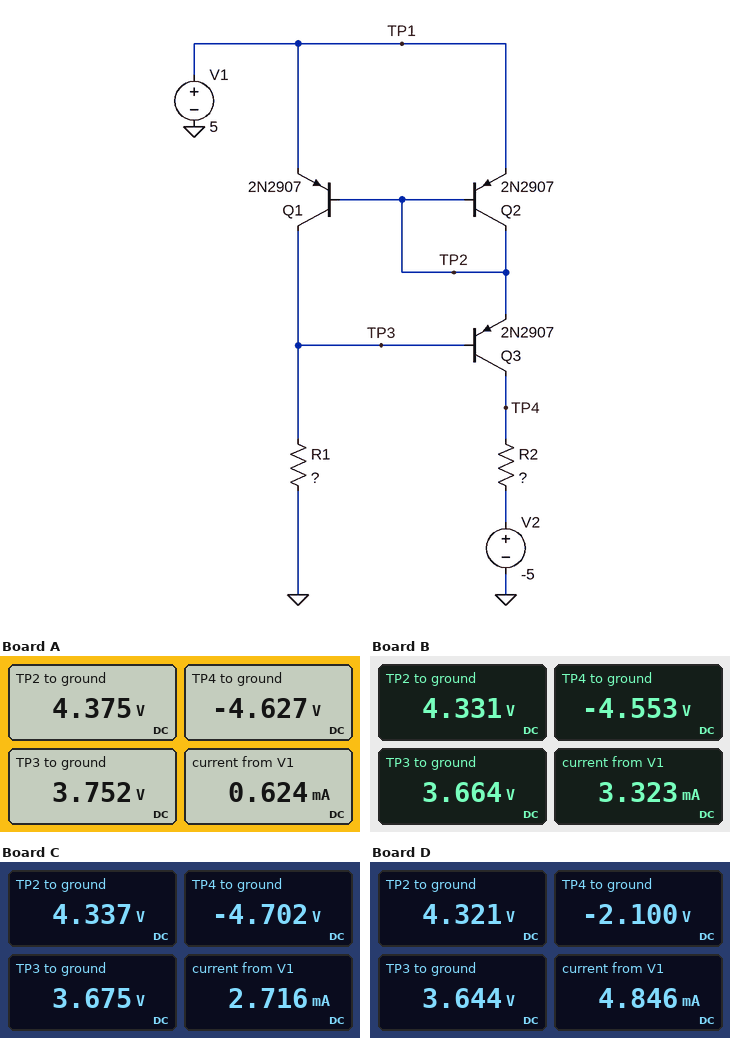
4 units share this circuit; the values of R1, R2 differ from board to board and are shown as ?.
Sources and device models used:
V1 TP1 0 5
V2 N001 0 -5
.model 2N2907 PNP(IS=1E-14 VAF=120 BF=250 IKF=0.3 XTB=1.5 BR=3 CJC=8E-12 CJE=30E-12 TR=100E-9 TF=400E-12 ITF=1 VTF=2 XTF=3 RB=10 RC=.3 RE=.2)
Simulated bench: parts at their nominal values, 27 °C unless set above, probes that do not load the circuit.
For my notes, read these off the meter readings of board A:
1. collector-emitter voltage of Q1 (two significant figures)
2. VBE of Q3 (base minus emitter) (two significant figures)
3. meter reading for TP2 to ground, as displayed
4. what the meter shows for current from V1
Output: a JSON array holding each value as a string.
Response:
["-1.2 V", "-620 mV", "4.375 V", "0.624 mA"]
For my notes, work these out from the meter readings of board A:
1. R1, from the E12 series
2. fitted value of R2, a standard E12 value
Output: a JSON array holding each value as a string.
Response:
["12 kΩ", "1.2 kΩ"]
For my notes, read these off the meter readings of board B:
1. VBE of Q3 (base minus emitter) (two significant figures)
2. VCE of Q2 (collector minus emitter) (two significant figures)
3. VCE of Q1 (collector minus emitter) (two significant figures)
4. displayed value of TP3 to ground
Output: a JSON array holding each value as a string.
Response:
["-670 mV", "-670 mV", "-1.3 V", "3.664 V"]
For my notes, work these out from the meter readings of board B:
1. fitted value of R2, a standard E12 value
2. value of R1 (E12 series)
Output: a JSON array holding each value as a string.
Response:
["270 Ω", "2.2 kΩ"]
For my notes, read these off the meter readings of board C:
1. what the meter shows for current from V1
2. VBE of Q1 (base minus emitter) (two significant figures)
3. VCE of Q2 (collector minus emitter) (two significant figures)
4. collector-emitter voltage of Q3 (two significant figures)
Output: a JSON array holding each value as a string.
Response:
["2.716 mA", "-660 mV", "-660 mV", "-9.0 V"]
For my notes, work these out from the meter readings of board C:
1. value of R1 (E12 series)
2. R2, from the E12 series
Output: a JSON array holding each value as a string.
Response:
["2.7 kΩ", "220 Ω"]
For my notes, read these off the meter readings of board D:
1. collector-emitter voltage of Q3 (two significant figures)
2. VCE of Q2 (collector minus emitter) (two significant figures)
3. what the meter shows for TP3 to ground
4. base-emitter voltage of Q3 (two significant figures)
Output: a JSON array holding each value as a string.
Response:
["-6.4 V", "-680 mV", "3.644 V", "-680 mV"]
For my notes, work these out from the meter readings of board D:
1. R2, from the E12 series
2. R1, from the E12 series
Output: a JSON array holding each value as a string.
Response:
["1.2 kΩ", "1.5 kΩ"]
